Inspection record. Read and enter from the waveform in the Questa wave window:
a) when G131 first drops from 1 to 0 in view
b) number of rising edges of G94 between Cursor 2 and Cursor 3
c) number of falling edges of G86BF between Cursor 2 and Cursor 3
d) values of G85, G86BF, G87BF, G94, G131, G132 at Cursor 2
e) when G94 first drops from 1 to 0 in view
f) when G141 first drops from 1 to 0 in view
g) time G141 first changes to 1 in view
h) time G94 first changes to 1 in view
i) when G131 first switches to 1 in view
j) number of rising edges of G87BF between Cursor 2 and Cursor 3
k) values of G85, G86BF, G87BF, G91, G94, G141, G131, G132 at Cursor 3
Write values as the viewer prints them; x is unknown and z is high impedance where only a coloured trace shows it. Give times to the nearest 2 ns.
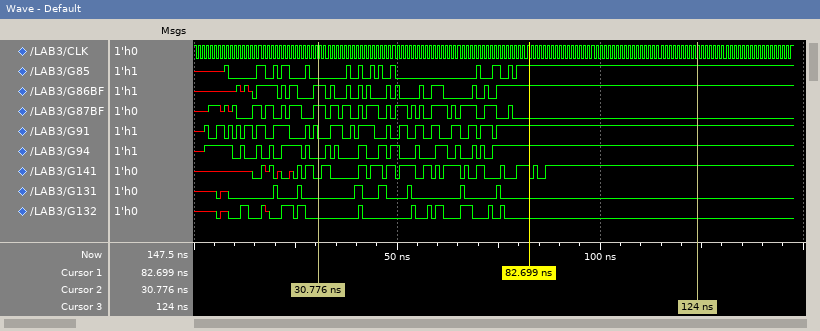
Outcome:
20 ns
11
11
G85=0, G86BF=1, G87BF=1, G94=0, G131=0, G132=0
10 ns
20 ns
16 ns
2 ns
20 ns
13
G85=1, G86BF=1, G87BF=0, G91=1, G94=1, G141=1, G131=0, G132=0
